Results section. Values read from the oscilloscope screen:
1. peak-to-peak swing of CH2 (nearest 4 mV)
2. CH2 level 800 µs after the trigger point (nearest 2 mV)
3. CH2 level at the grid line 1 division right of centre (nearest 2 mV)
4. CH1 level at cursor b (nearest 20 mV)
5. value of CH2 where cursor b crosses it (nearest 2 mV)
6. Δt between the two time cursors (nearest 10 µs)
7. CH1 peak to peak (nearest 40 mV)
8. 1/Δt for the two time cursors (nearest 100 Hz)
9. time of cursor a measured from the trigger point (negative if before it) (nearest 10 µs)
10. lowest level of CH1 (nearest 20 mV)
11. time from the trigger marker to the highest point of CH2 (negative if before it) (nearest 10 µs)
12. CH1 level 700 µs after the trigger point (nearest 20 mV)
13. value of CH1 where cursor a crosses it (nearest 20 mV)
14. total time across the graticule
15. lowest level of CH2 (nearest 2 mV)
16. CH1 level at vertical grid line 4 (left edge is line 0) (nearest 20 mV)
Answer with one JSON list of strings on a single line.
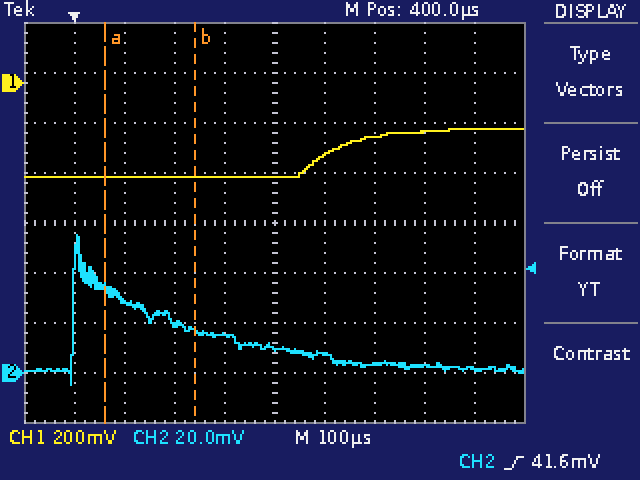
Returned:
["60 mV", "2 mV", "8 mV", "-380 mV", "16 mV", "180 µs", "200 mV", "5.6 kHz", "+60 µs", "-380 mV", "+10 µs", "-200 mV", "-380 mV", "1 ms", "-4 mV", "-380 mV"]
